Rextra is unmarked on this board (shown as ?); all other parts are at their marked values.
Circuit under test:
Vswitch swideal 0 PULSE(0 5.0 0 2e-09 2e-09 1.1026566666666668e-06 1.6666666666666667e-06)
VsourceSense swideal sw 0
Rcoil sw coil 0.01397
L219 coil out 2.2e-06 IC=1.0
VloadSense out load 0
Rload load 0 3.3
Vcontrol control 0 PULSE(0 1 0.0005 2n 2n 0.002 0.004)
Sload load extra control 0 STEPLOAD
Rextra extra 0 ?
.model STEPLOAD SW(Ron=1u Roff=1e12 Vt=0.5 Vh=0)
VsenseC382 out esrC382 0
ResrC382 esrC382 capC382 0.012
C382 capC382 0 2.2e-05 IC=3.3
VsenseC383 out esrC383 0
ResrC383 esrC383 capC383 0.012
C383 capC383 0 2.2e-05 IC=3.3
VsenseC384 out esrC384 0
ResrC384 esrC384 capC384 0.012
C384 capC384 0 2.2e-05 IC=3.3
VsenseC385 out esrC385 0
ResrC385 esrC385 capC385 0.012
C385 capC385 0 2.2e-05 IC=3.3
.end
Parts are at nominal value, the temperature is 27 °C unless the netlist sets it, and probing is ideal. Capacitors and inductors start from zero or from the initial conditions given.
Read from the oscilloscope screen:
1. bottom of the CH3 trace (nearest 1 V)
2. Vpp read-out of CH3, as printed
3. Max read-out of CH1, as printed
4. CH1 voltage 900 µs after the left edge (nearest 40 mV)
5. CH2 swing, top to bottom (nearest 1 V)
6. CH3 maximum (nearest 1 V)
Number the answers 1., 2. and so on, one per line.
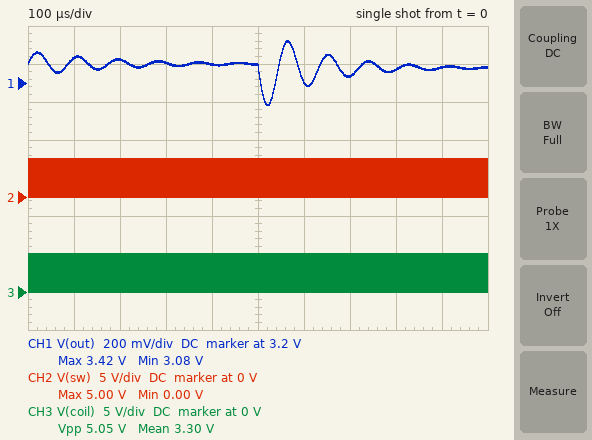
1. 0 V
2. 5.05 V
3. 3.42 V
4. 3.28 V
5. 5 V
6. 5 V
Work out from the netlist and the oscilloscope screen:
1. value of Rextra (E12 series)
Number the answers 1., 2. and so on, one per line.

1. 2.2 Ω
